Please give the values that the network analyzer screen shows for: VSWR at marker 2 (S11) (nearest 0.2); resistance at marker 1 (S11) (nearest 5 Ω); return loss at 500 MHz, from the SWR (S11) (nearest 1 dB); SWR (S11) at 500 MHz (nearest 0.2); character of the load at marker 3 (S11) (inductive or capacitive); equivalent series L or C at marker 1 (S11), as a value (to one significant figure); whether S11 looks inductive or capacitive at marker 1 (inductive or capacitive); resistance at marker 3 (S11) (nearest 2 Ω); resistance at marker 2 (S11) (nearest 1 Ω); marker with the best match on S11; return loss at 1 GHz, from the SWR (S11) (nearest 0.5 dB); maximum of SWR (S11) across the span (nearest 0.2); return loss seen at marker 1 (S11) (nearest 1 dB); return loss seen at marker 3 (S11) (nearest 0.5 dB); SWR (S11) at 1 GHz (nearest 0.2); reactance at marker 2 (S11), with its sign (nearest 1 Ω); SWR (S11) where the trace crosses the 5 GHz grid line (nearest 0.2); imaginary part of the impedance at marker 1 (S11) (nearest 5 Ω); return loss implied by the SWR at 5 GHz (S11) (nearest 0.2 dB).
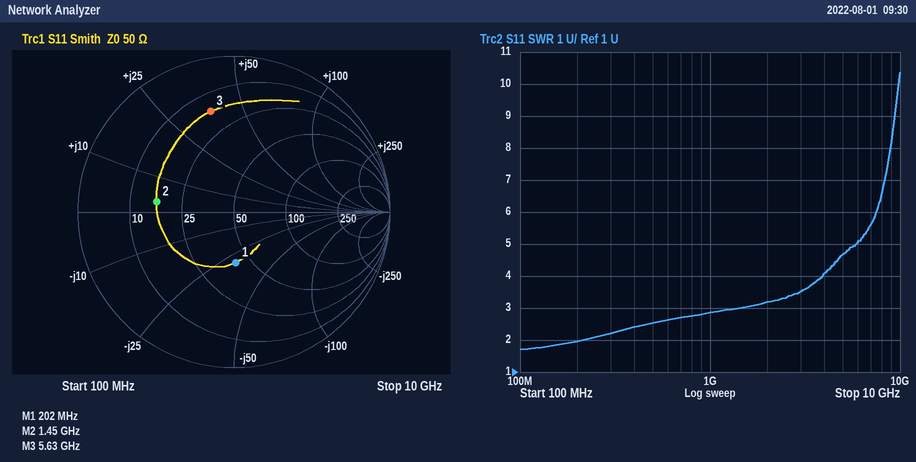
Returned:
3.0
40 Ω
7 dB
2.6
inductive
30 pF
capacitive
16 Ω
17 Ω
marker 1
6.5 dB
10.4
10 dB
3.5 dB
2.8
+3 Ω
4.6
-30 Ω
3.8 dB
